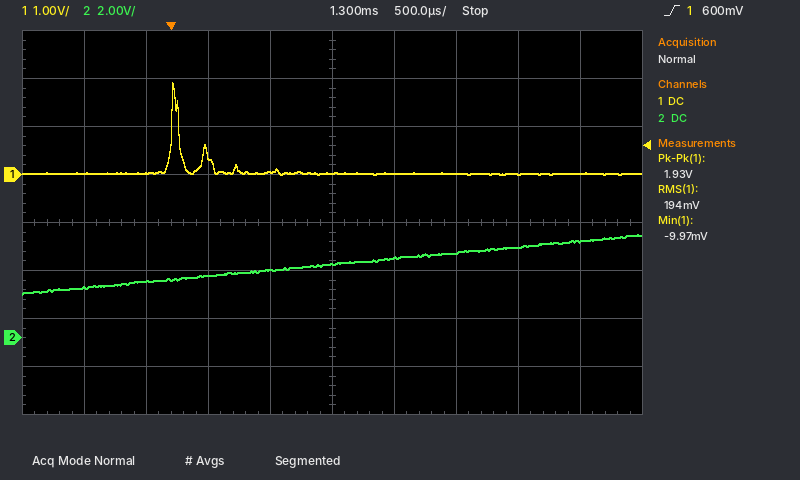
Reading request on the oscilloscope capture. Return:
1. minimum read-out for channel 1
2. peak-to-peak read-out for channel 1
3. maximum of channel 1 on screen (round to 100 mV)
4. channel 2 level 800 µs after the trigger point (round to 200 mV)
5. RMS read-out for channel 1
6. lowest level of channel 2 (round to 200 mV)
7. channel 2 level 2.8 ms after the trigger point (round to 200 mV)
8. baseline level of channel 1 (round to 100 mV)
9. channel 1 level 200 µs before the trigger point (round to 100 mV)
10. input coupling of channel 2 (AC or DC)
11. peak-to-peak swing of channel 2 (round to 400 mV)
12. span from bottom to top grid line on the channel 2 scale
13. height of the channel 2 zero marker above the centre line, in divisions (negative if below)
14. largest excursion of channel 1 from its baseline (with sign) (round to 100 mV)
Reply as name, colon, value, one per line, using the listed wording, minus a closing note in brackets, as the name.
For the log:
minimum read-out for channel 1: -9.97 mV
peak-to-peak read-out for channel 1: 1.93 V
maximum of channel 1 on screen: 1.9 V
channel 2 level 800 µs after the trigger point: 2.8 V
RMS read-out for channel 1: 194 mV
lowest level of channel 2: 1.8 V
channel 2 level 2.8 ms after the trigger point: 3.8 V
baseline level of channel 1: 0.0 V
channel 1 level 200 µs before the trigger point: 0.0 V
input coupling of channel 2: DC
peak-to-peak swing of channel 2: 2.4 V
span from bottom to top grid line on the channel 2 scale: 16 V
height of the channel 2 zero marker above the centre line, in divisions: -2.4 div
largest excursion of channel 1 from its baseline (with sign): +1.9 V
